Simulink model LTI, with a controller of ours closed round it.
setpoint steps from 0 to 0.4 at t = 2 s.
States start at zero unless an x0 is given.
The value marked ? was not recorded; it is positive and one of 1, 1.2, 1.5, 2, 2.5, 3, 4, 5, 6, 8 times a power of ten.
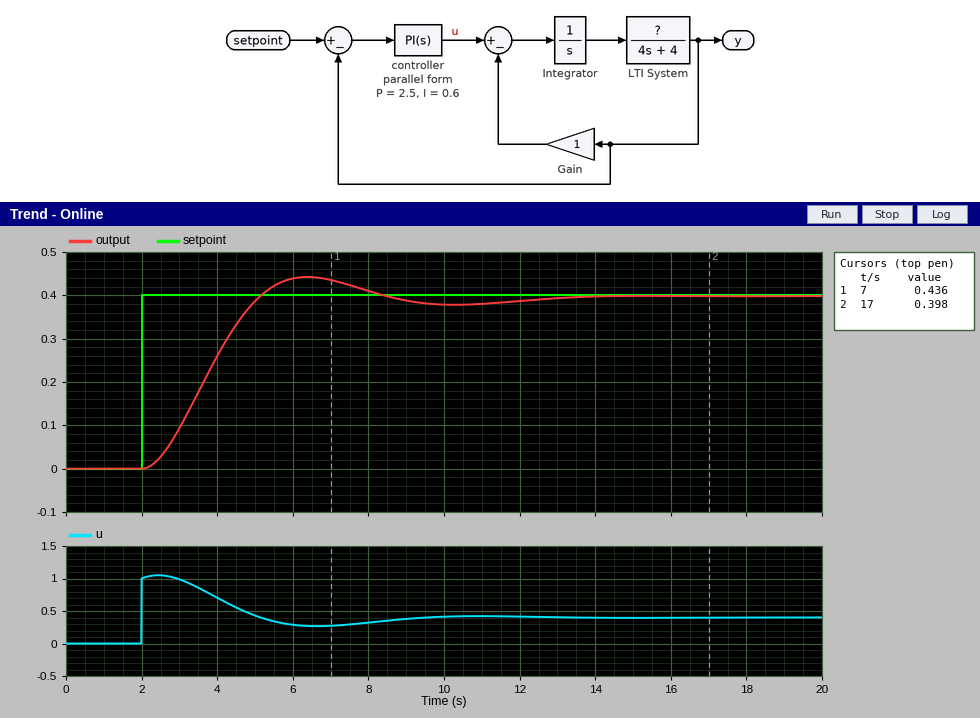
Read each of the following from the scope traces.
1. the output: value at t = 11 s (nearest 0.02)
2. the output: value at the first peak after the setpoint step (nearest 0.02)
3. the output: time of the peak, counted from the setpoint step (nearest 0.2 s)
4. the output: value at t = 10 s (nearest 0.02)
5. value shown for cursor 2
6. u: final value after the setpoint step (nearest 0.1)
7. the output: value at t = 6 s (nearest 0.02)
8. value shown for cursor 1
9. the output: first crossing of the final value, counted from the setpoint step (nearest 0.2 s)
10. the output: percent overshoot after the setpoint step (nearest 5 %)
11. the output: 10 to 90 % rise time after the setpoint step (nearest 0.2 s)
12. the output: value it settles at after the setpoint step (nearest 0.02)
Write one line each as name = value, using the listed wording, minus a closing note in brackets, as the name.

the output: value at t = 11 s = 0.38
the output: value at the first peak after the setpoint step = 0.44
the output: time of the peak, counted from the setpoint step = 4.4 s
the output: value at t = 10 s = 0.38
value shown for cursor 2 = 0.398
u: final value after the setpoint step = 0.4
the output: value at t = 6 s = 0.44
value shown for cursor 1 = 0.436
the output: first crossing of the final value, counted from the setpoint step = 3.2 s
the output: percent overshoot after the setpoint step = 10 %
the output: 10 to 90 % rise time after the setpoint step = 2.2 s
the output: value it settles at after the setpoint step = 0.40
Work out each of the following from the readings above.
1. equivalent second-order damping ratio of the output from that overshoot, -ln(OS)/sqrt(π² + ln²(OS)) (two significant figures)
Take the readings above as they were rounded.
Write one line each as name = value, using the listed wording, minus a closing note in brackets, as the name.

equivalent second-order damping ratio of the output from that overshoot, -ln(OS)/sqrt(π² + ln²(OS)) = 0.59
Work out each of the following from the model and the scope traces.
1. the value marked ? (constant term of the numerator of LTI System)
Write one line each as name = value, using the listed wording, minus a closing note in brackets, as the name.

the value marked ? = 1
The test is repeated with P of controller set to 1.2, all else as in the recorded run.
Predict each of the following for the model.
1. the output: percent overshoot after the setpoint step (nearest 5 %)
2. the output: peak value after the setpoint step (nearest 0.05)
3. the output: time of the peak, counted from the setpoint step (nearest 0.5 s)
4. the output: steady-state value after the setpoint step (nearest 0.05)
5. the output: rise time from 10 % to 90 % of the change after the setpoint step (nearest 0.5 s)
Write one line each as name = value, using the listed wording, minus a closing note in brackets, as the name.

the output: percent overshoot after the setpoint step = 20 %
the output: peak value after the setpoint step = 0.50
the output: time of the peak, counted from the setpoint step = 6.5 s
the output: steady-state value after the setpoint step = 0.40
the output: rise time from 10 % to 90 % of the change after the setpoint step = 3.0 s
